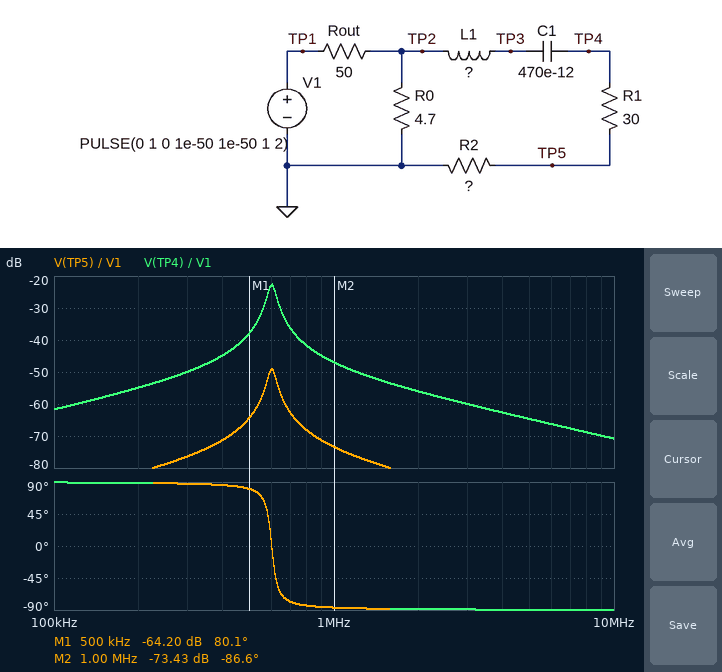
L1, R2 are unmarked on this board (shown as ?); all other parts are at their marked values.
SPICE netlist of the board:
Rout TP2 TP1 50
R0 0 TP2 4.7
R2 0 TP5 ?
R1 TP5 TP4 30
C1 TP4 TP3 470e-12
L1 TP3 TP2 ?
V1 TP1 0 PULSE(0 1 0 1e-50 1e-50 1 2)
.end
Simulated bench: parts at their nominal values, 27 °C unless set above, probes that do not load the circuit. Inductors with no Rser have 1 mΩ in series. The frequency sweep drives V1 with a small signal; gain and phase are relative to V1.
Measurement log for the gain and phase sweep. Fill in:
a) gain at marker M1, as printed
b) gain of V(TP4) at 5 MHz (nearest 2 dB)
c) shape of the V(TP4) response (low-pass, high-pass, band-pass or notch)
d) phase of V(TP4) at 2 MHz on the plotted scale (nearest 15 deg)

-64.20 dB
-64 dB
band-pass
-90 deg
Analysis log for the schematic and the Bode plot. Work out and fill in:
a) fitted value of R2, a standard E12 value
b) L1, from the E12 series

1.5 Ω
150 µH
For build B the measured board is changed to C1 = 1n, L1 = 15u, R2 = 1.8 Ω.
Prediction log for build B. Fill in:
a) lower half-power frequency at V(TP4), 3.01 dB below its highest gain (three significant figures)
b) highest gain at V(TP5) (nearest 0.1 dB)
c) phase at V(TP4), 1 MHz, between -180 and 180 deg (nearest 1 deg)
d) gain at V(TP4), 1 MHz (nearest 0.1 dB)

1.12 MHz
-47.4 dB
61 deg
-28.7 dB
